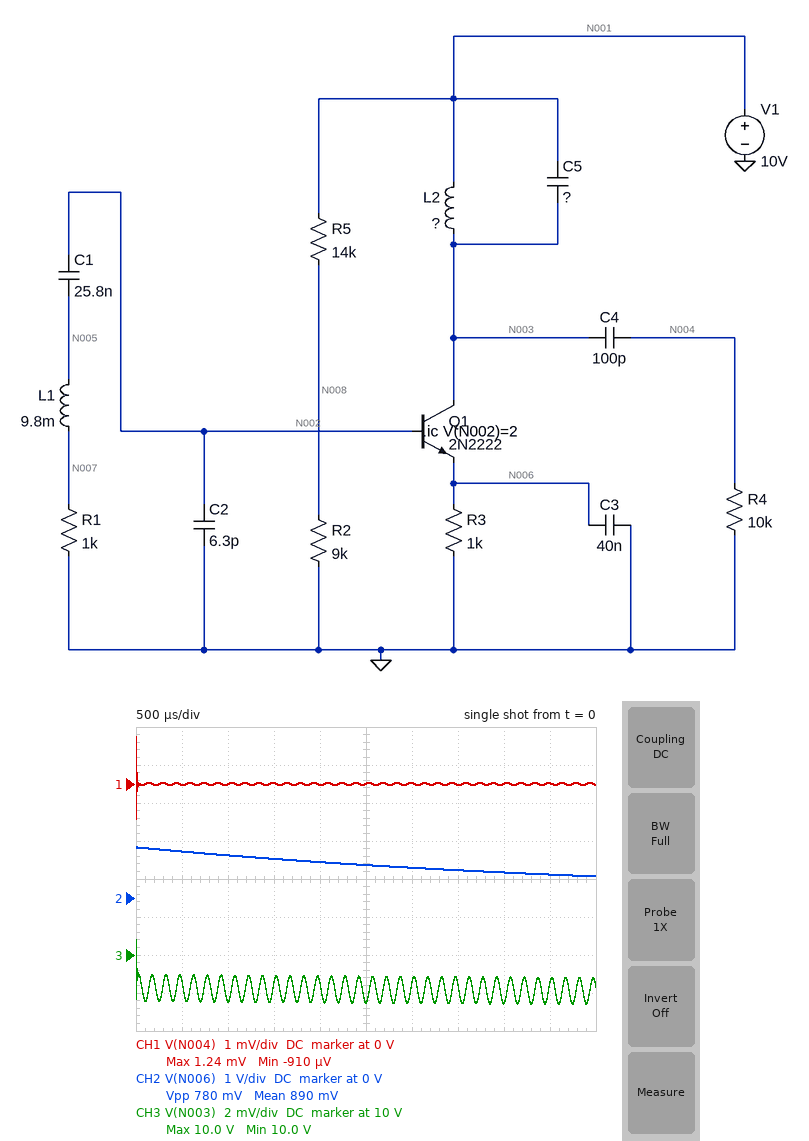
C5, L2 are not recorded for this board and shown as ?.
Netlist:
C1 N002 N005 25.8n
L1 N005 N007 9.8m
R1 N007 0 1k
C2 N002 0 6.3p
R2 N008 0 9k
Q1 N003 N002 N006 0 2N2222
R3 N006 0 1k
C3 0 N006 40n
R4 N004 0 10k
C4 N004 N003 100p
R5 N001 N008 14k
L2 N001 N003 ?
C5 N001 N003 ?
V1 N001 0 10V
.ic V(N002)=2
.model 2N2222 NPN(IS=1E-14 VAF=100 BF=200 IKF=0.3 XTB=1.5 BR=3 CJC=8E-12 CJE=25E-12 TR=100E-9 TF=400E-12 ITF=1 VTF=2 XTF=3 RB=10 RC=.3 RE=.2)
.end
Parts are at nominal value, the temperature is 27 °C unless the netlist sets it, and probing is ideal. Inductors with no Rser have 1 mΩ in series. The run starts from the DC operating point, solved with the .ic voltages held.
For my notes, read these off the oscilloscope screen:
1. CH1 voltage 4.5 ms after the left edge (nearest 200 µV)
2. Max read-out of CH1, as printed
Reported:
0 V
1.24 mV
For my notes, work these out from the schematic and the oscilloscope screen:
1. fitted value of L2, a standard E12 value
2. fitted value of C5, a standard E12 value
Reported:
1.2 mH
470 nF
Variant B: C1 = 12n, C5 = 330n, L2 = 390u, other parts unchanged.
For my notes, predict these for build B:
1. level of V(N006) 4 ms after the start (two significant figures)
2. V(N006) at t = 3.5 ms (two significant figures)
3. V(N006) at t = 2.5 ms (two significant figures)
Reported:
320 mV
380 mV
540 mV
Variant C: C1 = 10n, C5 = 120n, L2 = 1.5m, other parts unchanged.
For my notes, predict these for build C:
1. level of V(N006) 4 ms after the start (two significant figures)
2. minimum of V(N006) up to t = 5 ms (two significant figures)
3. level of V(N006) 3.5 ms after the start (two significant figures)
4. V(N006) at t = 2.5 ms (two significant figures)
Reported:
240 mV
160 mV
300 mV
450 mV
